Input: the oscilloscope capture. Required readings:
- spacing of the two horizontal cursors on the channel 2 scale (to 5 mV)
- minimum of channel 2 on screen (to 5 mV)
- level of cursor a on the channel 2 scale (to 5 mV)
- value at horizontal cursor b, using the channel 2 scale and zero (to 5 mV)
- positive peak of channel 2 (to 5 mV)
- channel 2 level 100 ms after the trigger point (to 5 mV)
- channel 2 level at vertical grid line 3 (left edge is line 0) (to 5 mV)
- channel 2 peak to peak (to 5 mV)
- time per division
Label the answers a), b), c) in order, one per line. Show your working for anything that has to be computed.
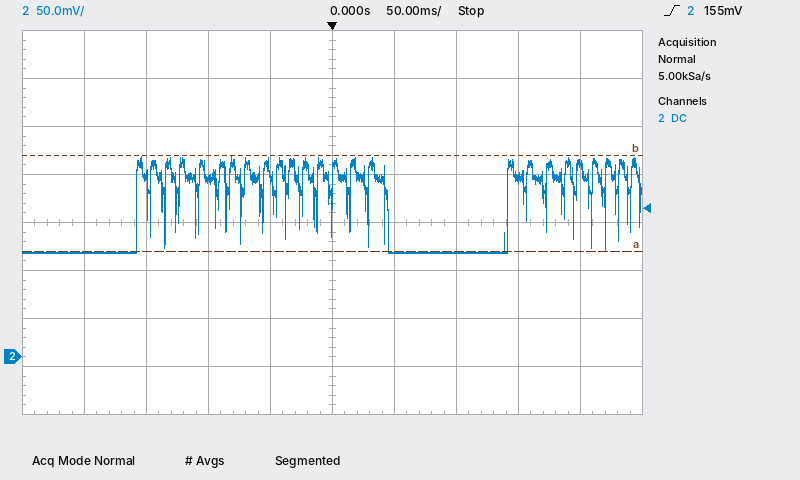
a) 100 mV
b) 110 mV
c) 110 mV
d) 210 mV
e) 210 mV
f) 110 mV
g) 185 mV
h) 210 mV − (110 mV) = 100 mV
i) 50 ms
